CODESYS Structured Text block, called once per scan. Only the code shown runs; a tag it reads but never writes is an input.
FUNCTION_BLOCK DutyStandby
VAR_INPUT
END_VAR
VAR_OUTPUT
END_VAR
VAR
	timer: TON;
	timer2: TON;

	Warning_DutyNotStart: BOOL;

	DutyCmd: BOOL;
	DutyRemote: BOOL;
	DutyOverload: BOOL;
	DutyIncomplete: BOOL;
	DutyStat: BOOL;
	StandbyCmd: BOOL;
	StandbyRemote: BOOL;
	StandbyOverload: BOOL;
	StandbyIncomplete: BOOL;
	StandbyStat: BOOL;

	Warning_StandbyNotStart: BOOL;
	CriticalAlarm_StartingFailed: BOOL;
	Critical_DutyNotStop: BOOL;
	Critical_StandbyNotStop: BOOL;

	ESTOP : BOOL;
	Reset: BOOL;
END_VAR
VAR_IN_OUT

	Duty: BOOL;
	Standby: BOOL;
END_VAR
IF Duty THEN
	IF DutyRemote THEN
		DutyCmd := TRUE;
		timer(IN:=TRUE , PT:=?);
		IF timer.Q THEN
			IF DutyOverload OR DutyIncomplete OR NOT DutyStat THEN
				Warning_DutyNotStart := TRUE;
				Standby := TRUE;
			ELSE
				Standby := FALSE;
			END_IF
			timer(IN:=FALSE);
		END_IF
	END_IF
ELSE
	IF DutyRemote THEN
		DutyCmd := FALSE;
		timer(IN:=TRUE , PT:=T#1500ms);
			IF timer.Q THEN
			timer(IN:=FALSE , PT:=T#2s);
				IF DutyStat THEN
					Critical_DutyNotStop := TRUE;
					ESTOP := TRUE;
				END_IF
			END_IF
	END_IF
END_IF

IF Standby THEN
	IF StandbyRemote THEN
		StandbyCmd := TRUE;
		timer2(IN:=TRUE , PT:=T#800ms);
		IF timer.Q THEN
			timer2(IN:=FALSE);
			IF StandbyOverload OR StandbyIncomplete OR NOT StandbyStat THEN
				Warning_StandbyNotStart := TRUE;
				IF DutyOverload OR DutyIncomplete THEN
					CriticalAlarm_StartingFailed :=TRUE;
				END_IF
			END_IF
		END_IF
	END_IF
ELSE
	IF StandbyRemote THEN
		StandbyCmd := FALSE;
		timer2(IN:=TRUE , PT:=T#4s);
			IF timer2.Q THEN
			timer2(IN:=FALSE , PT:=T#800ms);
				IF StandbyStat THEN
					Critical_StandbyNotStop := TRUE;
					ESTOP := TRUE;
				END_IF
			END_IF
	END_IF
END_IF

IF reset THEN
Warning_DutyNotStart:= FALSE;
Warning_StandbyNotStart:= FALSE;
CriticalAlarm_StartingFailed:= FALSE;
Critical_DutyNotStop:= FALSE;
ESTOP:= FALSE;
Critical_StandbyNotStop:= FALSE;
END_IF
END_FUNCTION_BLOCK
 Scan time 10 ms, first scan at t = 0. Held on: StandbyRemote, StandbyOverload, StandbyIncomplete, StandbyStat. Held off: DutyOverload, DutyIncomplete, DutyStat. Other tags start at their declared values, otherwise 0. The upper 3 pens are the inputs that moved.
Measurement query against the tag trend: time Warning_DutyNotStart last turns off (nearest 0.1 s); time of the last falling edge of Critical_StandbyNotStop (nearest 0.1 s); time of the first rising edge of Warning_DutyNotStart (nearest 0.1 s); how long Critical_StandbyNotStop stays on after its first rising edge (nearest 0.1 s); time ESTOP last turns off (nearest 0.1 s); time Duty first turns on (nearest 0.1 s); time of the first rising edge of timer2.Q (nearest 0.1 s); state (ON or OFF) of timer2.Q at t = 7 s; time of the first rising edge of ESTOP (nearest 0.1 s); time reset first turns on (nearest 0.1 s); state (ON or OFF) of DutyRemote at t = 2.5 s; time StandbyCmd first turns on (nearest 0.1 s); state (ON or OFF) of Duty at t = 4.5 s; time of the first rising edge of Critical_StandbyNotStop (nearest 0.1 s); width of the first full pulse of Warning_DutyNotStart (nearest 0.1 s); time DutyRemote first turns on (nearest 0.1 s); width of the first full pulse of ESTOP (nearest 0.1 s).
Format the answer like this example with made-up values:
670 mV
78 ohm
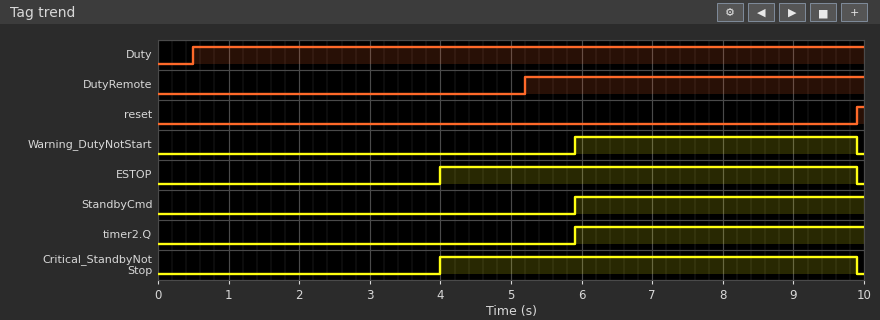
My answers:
9.9 s
9.9 s
5.9 s
5.9 s
9.9 s
0.5 s
5.9 s
ON
4.0 s
9.9 s
OFF
5.9 s
ON
4.0 s
4.0 s
5.2 s
5.9 s
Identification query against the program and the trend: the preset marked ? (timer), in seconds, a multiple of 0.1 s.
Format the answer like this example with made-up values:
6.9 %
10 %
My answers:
0.7 s
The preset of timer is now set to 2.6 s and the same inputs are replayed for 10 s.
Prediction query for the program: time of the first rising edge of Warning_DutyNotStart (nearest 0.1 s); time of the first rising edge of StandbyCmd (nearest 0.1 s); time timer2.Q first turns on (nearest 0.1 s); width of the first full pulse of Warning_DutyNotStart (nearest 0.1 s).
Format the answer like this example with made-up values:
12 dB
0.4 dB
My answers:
7.8 s
7.8 s
7.8 s
2.1 s
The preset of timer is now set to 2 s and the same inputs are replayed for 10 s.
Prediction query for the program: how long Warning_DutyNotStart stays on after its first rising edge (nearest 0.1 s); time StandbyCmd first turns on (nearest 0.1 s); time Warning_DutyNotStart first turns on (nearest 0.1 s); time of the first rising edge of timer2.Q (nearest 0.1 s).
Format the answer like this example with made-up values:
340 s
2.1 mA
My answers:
2.7 s
7.2 s
7.2 s
7.2 s
